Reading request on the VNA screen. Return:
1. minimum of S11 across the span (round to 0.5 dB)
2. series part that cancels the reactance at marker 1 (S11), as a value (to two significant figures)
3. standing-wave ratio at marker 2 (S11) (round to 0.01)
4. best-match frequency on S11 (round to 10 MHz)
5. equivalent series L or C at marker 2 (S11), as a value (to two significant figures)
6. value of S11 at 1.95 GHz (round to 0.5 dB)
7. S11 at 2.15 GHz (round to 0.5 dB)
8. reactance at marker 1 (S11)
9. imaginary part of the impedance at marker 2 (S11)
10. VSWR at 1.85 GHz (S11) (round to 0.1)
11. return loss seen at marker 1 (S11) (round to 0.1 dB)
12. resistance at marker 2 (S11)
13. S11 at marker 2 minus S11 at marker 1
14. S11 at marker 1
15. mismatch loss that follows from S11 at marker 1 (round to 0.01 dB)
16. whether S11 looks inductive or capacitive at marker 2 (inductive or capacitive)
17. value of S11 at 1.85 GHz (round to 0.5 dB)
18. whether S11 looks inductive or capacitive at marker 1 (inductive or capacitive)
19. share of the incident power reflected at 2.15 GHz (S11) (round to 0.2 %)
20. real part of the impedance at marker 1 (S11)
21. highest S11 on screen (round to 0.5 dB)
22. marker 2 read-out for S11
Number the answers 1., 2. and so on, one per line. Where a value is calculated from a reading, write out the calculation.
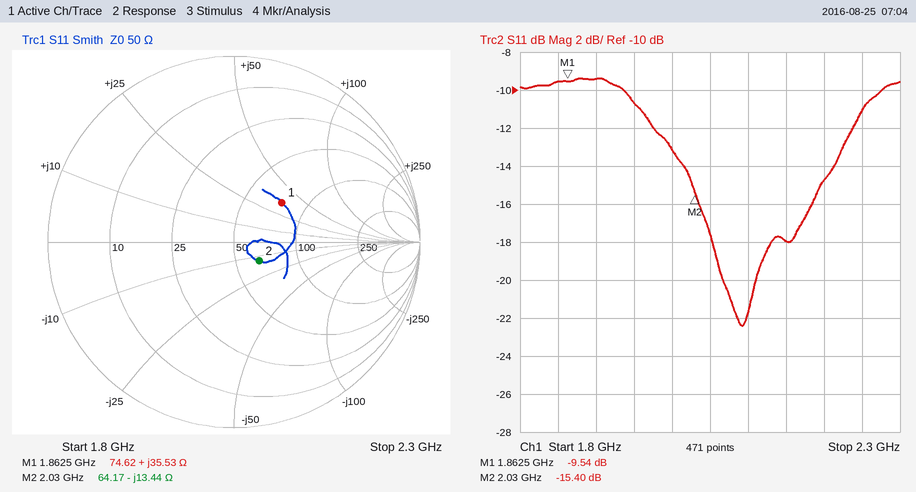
1. -22.5 dB
2. C = 1/(2π × 1.8625 GHz × 35.53 Ω) ≈ 2.4 pF
3. 1.41
4. 2.09 GHz
5. C = 1/(2π × 2.03 GHz × 13.44 Ω) ≈ 5.8 pF
6. -10.5 dB
7. -18.0 dB
8. +35.53 Ω
9. -13.44 Ω
10. |Γ| = 10^(-9.5/20) = 0.3350; VSWR = (1 + 0.3350)/(1 − 0.3350) ≈ 2.0
11. 9.5 dB
12. 64.17 Ω
13. -15.4 − (-9.54) = -5.86 dB
14. -9.54 dB
15. −10 log10(1 − 10^(-9.54/10)) ≈ 0.51 dB
16. capacitive
17. -9.5 dB
18. inductive
19. 10^(-18/10) ≈ 1.6 %
20. 74.62 Ω
21. -9.5 dB
22. -15.40 dB
